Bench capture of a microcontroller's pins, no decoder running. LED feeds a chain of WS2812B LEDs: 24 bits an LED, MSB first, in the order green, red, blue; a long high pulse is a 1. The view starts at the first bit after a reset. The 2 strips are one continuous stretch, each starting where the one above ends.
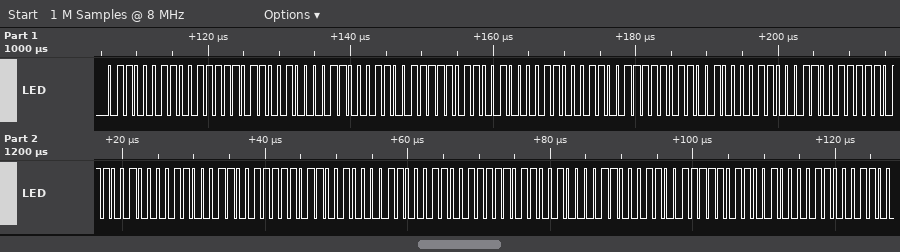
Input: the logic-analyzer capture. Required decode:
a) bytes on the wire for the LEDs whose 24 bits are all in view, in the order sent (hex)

63 3E C8 63 3E C8 63 3E C8 63 3E C8 63 3E C8 63 3E C8 63 3E C8
